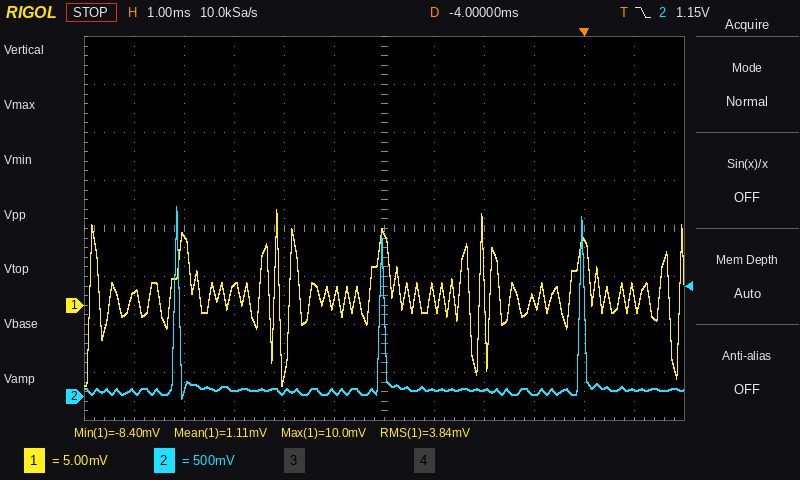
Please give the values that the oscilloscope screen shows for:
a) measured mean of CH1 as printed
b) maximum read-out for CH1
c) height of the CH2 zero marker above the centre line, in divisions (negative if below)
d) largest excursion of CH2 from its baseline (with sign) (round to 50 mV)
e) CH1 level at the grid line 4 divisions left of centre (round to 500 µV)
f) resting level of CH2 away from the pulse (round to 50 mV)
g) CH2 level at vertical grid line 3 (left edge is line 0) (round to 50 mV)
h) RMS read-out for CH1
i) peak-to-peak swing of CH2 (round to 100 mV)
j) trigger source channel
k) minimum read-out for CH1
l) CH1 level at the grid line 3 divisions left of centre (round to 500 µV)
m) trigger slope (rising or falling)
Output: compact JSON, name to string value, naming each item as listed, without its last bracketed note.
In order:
{"measured mean of CH1 as printed": "1.11 mV", "maximum read-out for CH1": "10.0 mV", "height of the CH2 zero marker above the centre line, in divisions": "-3.5 div", "largest excursion of CH2 from its baseline (with sign)": "+1.90 V", "CH1 level at the grid line 4 divisions left of centre": "7.0 mV", "resting level of CH2 away from the pulse": "50 mV", "CH2 level at vertical grid line 3 (left edge is line 0)": "50 mV", "RMS read-out for CH1": "3.84 mV", "peak-to-peak swing of CH2": "2.00 V", "trigger source channel": "CH2", "minimum read-out for CH1": "-8.40 mV", "CH1 level at the grid line 3 divisions left of centre": "2.0 mV", "trigger slope": "falling"}
